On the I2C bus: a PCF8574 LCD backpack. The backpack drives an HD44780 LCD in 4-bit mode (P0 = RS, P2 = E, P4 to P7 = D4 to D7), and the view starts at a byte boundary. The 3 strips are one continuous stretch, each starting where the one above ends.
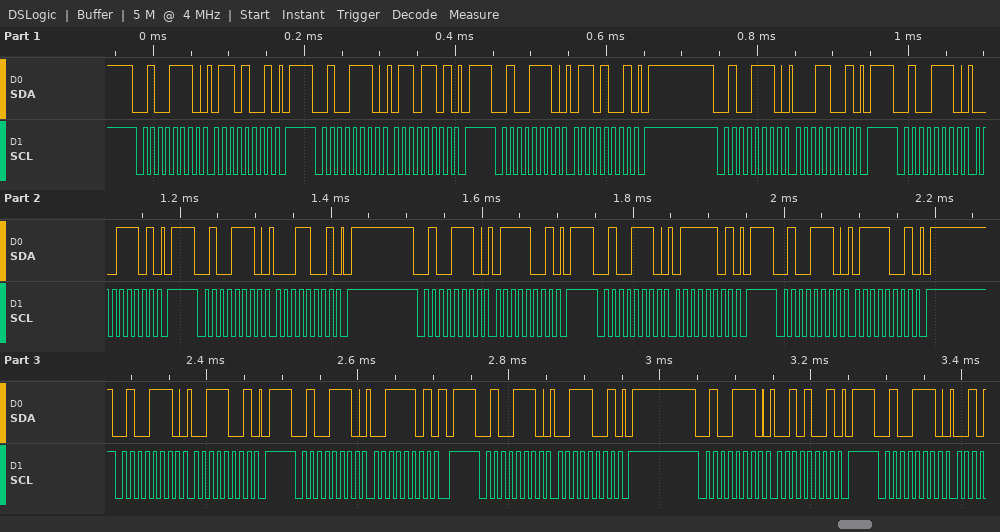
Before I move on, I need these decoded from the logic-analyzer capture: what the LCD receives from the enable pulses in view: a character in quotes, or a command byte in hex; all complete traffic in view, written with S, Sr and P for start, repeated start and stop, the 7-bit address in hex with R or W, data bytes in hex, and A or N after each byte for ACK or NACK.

'a' 's'
S 27W A 69 A P S 27W A 6D A P S 27W A 69 A P S 27W A 19 A P S 27W A 1D A P S 27W A 19 A P S 27W A 79 A P S 27W A 7D A P S 27W A 79 A P S 27W A 39 A P S 27W A 3D A P S 27W A 39 A P S 27W A 29 A P S 27W A
